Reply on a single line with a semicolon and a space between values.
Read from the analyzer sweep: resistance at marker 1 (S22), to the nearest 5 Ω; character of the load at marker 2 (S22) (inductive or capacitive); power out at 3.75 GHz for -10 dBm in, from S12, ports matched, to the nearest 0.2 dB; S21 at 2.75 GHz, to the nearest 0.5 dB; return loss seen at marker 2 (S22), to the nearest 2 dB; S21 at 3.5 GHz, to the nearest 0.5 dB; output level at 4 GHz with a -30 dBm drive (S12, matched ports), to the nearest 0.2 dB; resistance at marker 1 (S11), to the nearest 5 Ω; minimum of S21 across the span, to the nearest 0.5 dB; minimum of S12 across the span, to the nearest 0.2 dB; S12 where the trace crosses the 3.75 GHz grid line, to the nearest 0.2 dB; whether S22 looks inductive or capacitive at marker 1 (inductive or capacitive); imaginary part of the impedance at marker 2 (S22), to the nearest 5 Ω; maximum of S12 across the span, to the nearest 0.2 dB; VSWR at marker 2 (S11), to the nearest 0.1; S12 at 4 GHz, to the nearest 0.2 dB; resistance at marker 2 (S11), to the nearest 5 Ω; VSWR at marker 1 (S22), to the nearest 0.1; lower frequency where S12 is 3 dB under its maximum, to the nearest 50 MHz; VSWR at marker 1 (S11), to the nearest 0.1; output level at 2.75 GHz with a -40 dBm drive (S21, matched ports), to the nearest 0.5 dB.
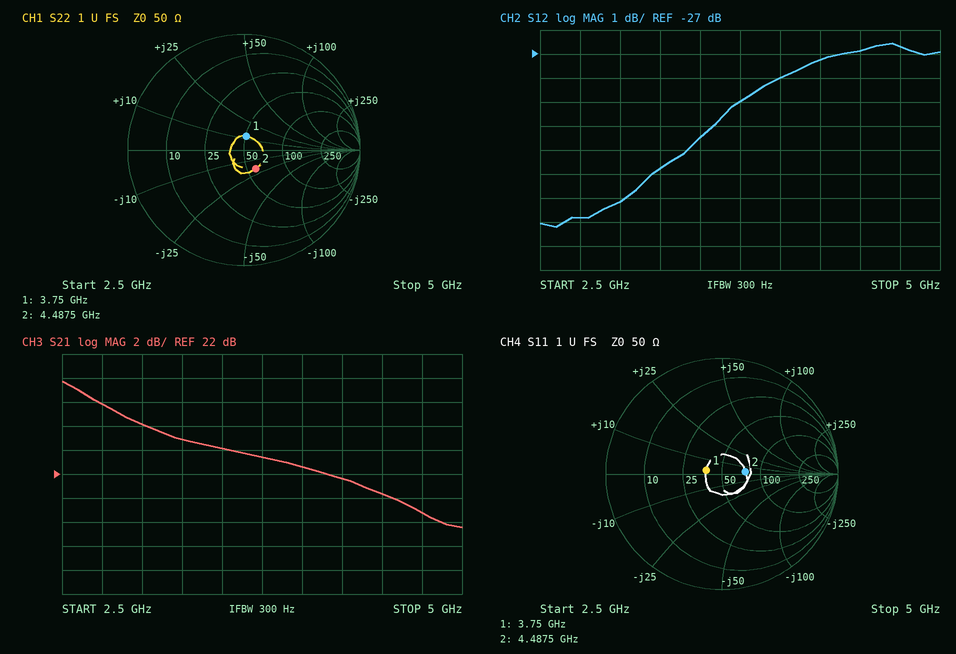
50 Ω; capacitive; -39.0 dBm; 28.0 dB; 14 dB; 24.0 dB; -58.0 dBm; 40 Ω; 17.5 dB; -34.2 dB; -29.0 dB; inductive; -20 Ω; -26.6 dB; 1.5; -28.0 dB; 75 Ω; 1.3; 3.65 GHz; 1.3; -12.0 dBm
